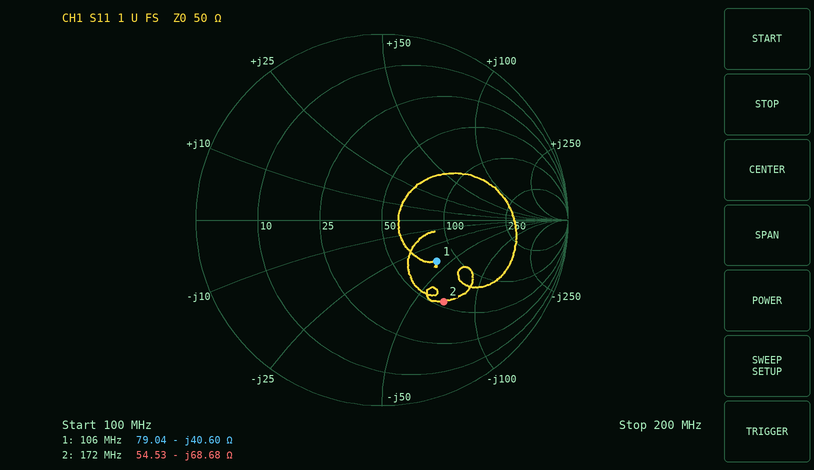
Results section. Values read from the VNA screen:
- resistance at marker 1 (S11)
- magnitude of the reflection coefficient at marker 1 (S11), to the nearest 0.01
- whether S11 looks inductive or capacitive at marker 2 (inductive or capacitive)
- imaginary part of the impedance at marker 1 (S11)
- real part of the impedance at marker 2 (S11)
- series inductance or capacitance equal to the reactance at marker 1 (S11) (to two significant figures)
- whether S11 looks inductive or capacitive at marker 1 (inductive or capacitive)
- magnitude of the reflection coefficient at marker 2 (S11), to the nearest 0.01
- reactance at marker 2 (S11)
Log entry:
79.04 Ω
0.37
capacitive
-40.60 Ω
54.53 Ω
37 pF
capacitive
0.55
-68.68 Ω
